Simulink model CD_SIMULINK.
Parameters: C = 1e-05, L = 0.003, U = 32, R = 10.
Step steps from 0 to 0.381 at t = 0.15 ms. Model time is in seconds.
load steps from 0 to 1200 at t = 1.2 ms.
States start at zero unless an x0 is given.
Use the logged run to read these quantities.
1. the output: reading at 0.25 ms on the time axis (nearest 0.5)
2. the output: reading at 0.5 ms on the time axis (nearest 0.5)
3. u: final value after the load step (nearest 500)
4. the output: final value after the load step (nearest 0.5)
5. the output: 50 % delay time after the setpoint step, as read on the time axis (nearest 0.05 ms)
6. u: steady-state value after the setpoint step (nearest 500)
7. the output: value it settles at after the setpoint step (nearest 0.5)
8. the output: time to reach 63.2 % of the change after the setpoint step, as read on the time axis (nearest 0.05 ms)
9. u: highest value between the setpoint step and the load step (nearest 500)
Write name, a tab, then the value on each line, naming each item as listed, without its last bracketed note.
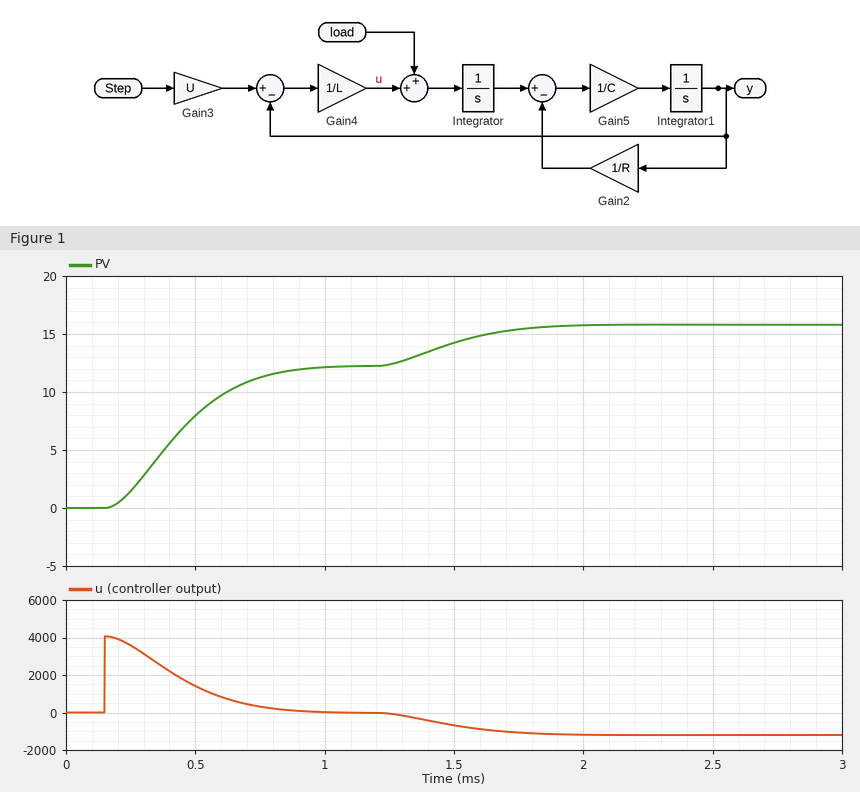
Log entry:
the output: reading at 0.25 ms on the time axis	1.5
the output: reading at 0.5 ms on the time axis	8.0
u: final value after the load step	-1000
the output: final value after the load step	16.0
the output: 50 % delay time after the setpoint step, as read on the time axis	0.40 ms
u: steady-state value after the setpoint step	0
the output: value it settles at after the setpoint step	12.0
the output: time to reach 63.2 % of the change after the setpoint step, as read on the time axis	0.50 ms
u: highest value between the setpoint step and the load step	4000
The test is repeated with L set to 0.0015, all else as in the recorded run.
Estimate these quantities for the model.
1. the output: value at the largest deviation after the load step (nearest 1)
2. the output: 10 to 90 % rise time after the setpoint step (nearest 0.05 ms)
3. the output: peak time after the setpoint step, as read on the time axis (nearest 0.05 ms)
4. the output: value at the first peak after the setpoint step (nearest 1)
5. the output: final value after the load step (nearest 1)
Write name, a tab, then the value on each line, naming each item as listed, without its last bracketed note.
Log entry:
the output: value at the largest deviation after the load step	14
the output: 10 to 90 % rise time after the setpoint step	0.25 ms
the output: peak time after the setpoint step, as read on the time axis	0.65 ms
the output: value at the first peak after the setpoint step	13
the output: final value after the load step	14
